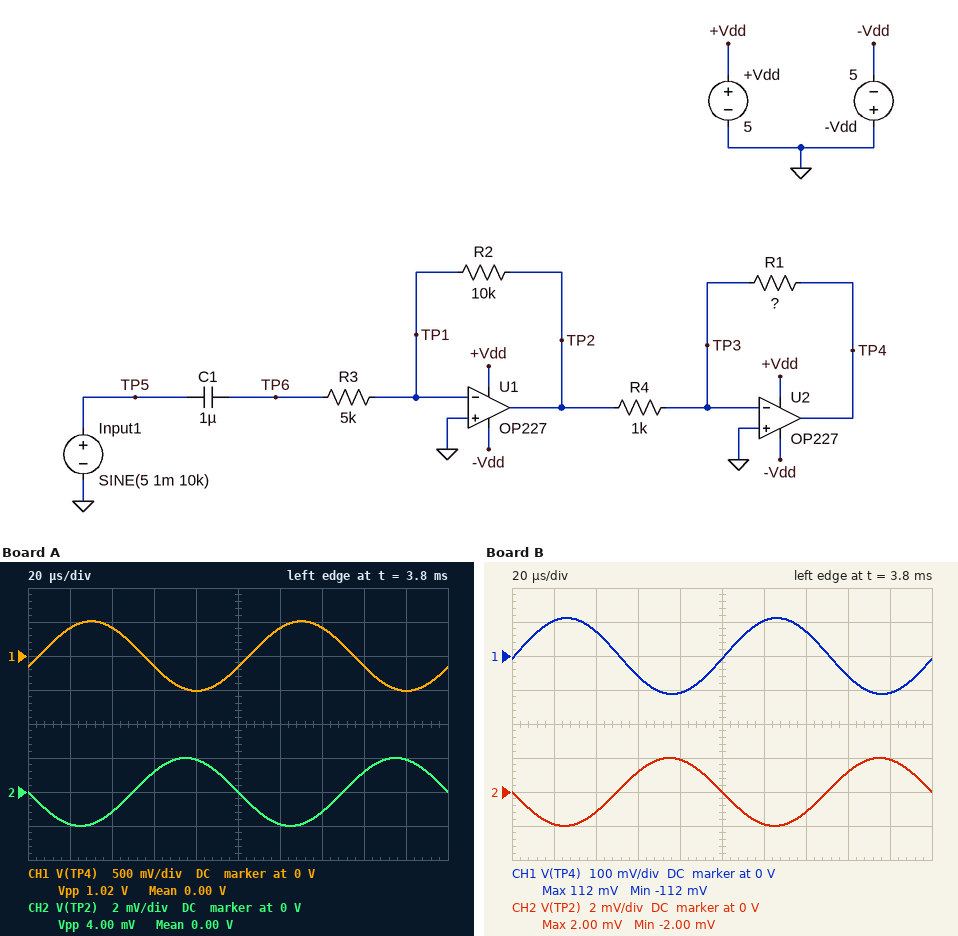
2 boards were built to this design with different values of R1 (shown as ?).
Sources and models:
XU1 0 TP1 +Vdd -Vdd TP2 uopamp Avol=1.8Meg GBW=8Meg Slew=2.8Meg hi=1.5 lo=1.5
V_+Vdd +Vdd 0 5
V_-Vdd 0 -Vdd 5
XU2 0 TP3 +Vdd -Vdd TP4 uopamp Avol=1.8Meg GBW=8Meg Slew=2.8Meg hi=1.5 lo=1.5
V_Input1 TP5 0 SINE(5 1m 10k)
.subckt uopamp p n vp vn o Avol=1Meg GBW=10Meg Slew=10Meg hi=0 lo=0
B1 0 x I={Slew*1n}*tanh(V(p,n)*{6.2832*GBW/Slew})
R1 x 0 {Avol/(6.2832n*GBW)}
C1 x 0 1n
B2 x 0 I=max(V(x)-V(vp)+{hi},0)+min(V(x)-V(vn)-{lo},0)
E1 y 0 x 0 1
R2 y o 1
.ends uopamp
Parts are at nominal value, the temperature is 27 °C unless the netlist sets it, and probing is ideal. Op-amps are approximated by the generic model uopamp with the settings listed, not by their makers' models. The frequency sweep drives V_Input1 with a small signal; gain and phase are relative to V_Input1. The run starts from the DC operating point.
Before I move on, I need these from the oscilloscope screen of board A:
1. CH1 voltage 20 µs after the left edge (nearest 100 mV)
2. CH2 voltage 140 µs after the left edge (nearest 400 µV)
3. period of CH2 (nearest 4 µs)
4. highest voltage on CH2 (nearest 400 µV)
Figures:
400 mV
-1.2 mV
100 µs
2.0 mV
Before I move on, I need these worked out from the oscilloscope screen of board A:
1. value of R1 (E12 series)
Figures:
270 kΩ
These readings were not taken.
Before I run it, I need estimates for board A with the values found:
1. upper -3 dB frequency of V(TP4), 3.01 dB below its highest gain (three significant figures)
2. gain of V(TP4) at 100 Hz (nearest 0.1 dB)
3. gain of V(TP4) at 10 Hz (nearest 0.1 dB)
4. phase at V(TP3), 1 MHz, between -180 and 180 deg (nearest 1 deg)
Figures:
29.6 kHz
54.2 dB
44.2 dB
161 deg
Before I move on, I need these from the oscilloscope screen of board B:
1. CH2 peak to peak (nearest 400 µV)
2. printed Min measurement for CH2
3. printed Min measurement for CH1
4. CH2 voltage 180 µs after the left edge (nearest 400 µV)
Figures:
4.0 mV
-2.00 mV
-112 mV
2.0 mV
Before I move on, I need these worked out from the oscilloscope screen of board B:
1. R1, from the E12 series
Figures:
56 kΩ
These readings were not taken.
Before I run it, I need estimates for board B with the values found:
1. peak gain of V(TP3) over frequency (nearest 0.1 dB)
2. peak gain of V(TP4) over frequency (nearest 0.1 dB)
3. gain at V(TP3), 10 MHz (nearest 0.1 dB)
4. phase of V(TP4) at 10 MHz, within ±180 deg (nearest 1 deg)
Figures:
5.4 dB
41.0 dB
-5.9 dB
-164 deg
